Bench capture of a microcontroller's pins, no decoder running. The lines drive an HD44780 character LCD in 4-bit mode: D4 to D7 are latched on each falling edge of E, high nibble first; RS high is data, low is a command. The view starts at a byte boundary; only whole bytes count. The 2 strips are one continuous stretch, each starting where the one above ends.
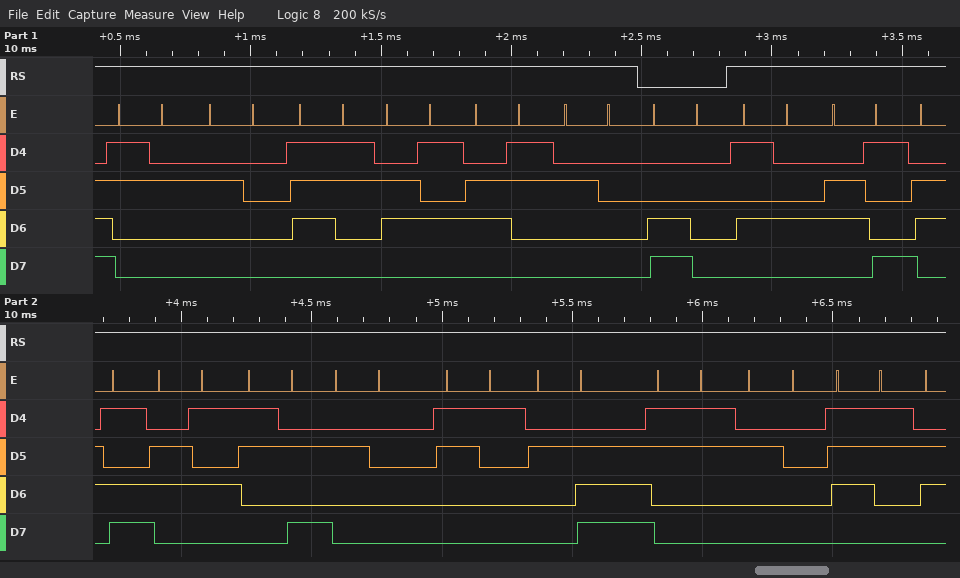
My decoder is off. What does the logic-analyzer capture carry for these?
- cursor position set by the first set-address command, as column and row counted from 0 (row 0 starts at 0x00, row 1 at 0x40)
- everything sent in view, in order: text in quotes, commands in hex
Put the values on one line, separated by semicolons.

column 0, row 1; "2 sec " 0xC0 "Time: 1.3 s"
